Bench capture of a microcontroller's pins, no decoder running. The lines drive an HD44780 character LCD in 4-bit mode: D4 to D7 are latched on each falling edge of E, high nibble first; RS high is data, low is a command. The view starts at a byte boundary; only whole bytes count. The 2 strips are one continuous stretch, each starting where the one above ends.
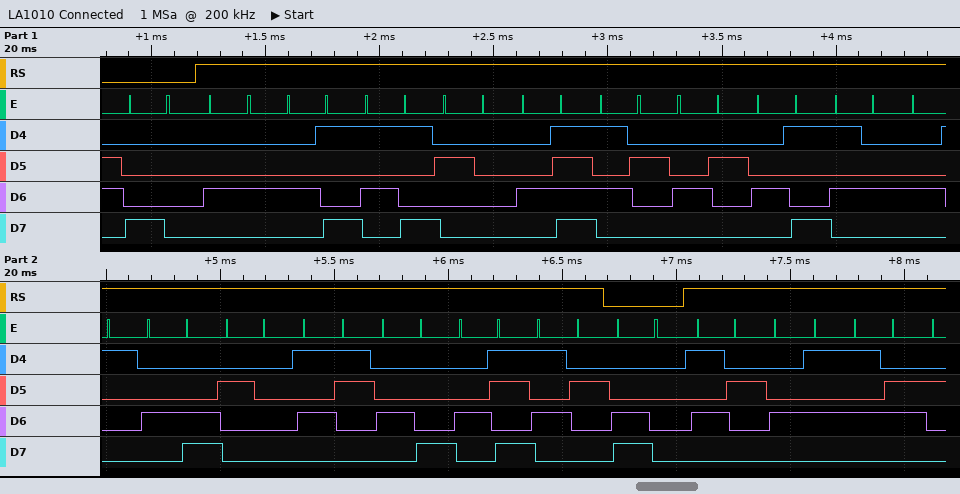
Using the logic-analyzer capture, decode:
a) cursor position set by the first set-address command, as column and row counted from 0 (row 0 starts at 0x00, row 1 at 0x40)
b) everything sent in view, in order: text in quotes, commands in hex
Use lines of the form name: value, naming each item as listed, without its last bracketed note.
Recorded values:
cursor position set by the first set-address command, as column and row counted from 0: column 0, row 0
everything sent in view, in order: text in quotes, commands in hex: 0x80 "DIY ORBITAL SHKR" 0xC0 "REV"
